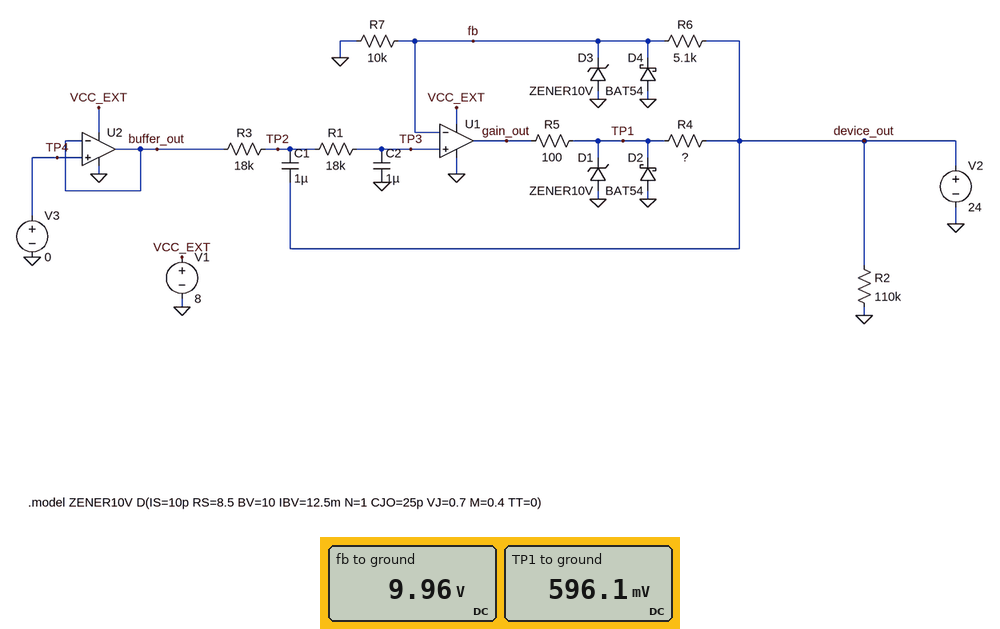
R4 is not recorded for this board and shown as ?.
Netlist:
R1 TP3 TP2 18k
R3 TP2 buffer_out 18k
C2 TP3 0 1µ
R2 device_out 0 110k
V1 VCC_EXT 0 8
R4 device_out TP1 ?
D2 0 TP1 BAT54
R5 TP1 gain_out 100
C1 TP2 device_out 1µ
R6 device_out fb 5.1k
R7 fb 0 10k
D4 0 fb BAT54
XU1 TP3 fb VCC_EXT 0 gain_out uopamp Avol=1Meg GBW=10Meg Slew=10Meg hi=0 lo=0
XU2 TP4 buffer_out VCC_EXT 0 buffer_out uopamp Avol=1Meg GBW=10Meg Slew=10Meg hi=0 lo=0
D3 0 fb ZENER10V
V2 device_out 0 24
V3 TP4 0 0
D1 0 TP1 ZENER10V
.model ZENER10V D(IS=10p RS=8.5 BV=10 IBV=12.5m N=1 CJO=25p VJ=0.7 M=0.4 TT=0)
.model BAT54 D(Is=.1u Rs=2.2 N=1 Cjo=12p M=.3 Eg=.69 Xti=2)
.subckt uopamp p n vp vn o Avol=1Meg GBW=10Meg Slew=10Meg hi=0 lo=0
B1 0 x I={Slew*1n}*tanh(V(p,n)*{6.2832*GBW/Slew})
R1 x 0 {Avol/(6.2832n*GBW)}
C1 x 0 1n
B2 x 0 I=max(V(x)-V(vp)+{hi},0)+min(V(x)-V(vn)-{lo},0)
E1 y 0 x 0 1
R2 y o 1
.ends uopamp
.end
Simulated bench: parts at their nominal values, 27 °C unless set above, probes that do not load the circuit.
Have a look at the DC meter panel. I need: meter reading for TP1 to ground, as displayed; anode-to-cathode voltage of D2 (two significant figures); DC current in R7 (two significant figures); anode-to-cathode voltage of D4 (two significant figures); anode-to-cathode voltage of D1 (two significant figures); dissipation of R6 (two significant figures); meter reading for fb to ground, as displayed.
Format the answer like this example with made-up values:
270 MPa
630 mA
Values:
596.1 mV
-600 mV
1.0 mA
-10 V
-600 mV
39 mW
9.96 V
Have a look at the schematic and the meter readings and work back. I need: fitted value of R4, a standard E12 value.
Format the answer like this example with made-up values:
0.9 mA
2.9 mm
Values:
3.9 kΩ
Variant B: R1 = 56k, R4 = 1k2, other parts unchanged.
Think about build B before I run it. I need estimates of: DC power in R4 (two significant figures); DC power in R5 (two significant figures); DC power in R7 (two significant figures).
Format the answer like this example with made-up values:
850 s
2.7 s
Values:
410 mW
34 mW
9.9 mW
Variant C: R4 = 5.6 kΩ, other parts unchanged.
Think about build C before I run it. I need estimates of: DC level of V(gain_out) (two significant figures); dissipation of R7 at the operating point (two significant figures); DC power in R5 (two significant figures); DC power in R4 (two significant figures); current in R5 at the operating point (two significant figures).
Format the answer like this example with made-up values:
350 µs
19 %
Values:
-5.8 mV
9.9 mW
1.8 mW
99 mW
4.2 mA
